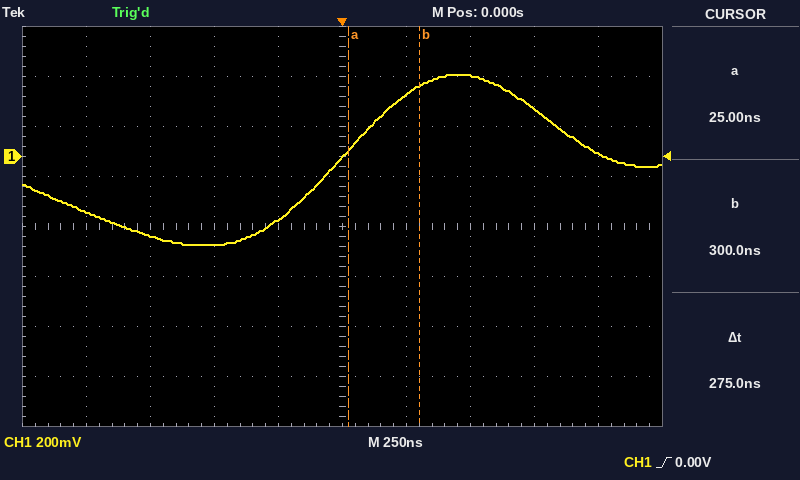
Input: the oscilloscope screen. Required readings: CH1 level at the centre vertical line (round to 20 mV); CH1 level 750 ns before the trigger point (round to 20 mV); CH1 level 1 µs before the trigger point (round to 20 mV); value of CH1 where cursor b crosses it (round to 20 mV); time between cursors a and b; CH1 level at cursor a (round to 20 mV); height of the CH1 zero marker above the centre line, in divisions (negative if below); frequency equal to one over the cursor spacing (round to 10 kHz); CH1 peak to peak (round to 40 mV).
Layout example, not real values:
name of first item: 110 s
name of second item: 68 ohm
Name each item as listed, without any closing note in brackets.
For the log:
CH1 level at the centre vertical line: 0 mV
CH1 level 750 ns before the trigger point: -320 mV
CH1 level 1 µs before the trigger point: -220 mV
value of CH1 where cursor b crosses it: 280 mV
time between cursors a and b: 275 ns
CH1 level at cursor a: 20 mV
height of the CH1 zero marker above the centre line, in divisions: +1.4 div
frequency equal to one over the cursor spacing: 3.64 MHz
CH1 peak to peak: 680 mV
